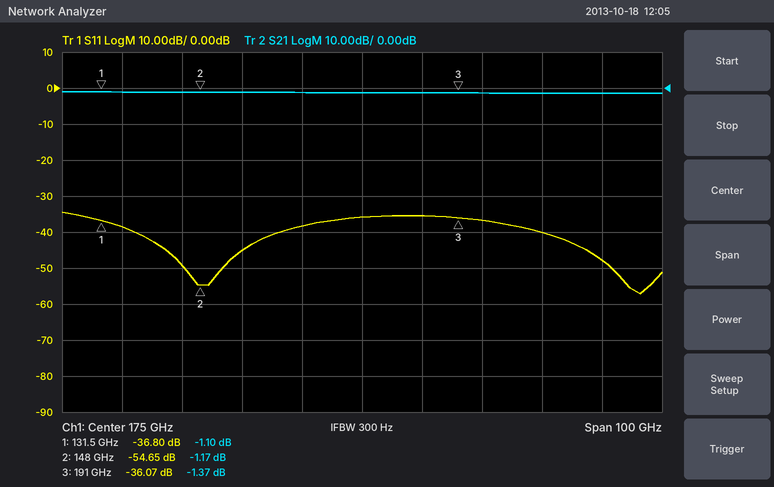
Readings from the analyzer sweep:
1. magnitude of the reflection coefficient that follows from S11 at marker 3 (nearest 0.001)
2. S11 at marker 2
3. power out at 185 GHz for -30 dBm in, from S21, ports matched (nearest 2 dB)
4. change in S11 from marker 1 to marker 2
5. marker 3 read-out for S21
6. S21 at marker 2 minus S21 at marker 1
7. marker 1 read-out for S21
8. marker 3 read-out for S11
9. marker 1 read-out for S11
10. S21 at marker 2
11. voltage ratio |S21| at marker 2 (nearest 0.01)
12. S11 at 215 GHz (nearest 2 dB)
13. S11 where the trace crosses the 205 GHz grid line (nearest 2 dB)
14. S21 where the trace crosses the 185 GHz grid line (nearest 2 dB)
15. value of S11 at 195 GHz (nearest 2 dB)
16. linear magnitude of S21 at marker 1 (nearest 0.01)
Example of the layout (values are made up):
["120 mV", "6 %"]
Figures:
["0.016", "-54.65 dB", "-32 dBm", "-17.85 dB", "-1.37 dB", "-0.07 dB", "-1.10 dB", "-36.07 dB", "-36.80 dB", "-1.17 dB", "0.87", "-48 dB", "-40 dB", "-2 dB", "-36 dB", "0.88"]
